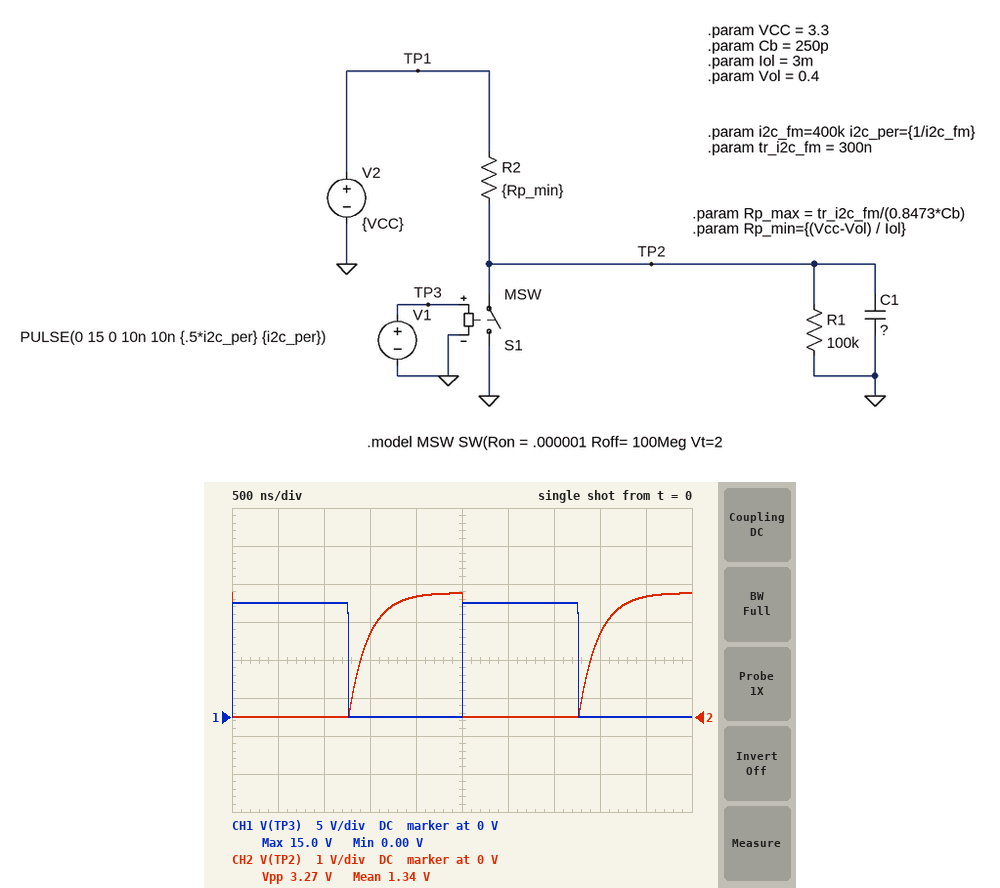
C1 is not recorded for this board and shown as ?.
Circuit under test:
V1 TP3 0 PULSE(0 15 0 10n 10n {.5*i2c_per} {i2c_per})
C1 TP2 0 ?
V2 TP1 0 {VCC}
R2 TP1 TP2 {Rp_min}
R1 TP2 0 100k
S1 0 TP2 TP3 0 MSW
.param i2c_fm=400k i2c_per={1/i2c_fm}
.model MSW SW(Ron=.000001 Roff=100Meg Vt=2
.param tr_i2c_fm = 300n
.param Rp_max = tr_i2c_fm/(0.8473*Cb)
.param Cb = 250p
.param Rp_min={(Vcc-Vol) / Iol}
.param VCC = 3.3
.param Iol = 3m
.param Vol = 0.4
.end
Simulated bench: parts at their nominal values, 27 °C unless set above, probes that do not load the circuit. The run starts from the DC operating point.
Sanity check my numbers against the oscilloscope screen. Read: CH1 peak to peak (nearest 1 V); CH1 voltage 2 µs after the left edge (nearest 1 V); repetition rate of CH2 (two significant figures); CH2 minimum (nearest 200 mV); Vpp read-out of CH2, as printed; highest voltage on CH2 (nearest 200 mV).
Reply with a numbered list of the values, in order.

1. 15 V
2. 0 V
3. 400 kHz
4. 0 V
5. 3.27 V
6. 3.2 V
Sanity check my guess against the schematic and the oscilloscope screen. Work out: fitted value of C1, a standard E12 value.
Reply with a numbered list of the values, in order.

1. 220 pF
